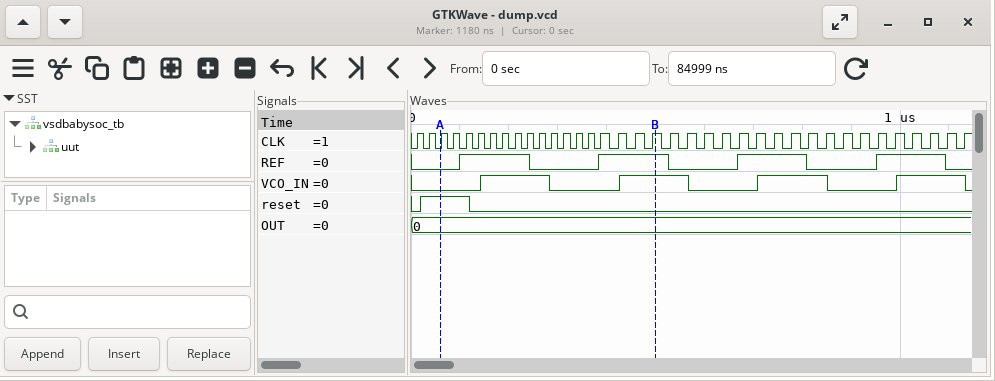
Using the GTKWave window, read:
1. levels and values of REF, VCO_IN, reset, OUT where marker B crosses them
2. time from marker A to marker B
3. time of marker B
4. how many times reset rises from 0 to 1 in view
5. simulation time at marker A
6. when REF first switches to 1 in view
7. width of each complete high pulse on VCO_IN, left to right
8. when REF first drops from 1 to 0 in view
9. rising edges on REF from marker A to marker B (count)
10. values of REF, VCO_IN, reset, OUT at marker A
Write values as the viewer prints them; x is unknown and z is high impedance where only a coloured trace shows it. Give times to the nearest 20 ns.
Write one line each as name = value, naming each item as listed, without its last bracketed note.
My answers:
levels and values of REF, VCO_IN, reset, OUT where marker B crosses them = REF=1, VCO_IN=1, reset=0, OUT=0
time from marker A to marker B = 440 ns
time of marker B = 500 ns
how many times reset rises from 0 to 1 in view = 1
simulation time at marker A = 60 ns
when REF first switches to 1 in view = 100 ns
width of each complete high pulse on VCO_IN, left to right = 140 ns, 140 ns, 140 ns, 140 ns
when REF first drops from 1 to 0 in view = 240 ns
rising edges on REF from marker A to marker B = 2
values of REF, VCO_IN, reset, OUT at marker A = REF=0, VCO_IN=0, reset=1, OUT=0
